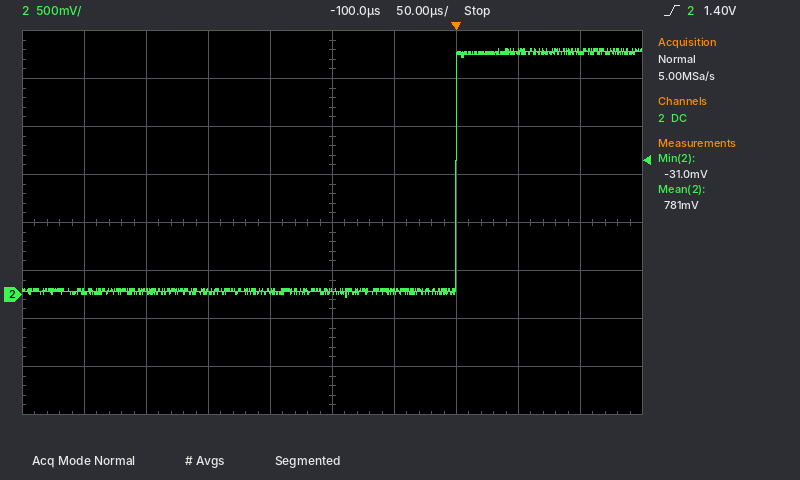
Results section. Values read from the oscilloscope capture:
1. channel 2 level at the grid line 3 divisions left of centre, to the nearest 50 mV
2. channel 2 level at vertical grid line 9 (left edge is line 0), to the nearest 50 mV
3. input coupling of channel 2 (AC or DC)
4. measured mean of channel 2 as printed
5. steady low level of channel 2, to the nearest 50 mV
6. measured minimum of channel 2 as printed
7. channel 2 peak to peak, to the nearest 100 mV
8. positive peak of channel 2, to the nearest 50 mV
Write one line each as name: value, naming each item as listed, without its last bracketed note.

channel 2 level at the grid line 3 divisions left of centre, to the nearest 50 mV: 50 mV
channel 2 level at vertical grid line 9 (left edge is line 0), to the nearest 50 mV: 2.55 V
input coupling of channel 2: DC
measured mean of channel 2 as printed: 781 mV
steady low level of channel 2, to the nearest 50 mV: 50 mV
measured minimum of channel 2 as printed: -31.0 mV
channel 2 peak to peak, to the nearest 100 mV: 2.60 V
positive peak of channel 2, to the nearest 50 mV: 2.55 V
